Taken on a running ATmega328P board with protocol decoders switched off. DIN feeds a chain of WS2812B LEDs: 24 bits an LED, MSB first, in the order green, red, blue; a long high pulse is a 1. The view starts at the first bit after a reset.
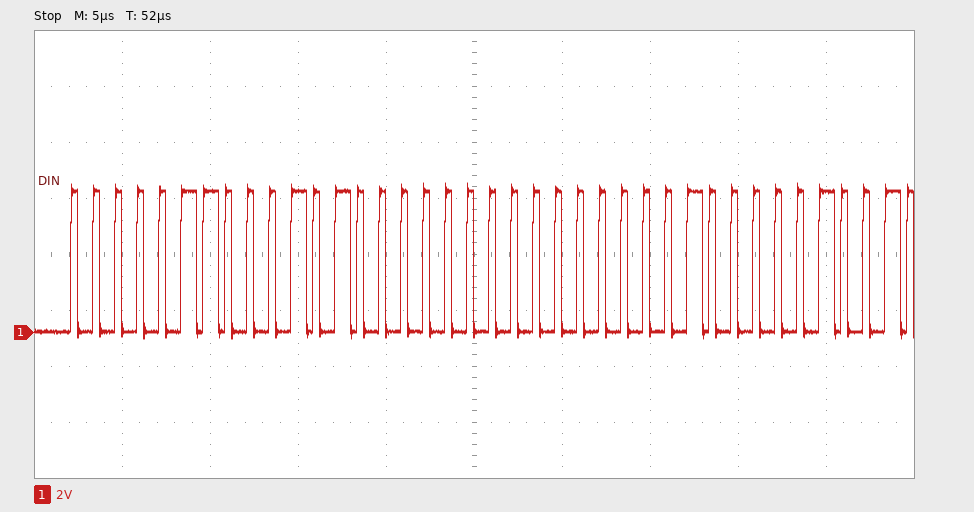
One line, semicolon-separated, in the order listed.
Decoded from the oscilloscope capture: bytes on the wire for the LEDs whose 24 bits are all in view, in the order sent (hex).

06 28 00
